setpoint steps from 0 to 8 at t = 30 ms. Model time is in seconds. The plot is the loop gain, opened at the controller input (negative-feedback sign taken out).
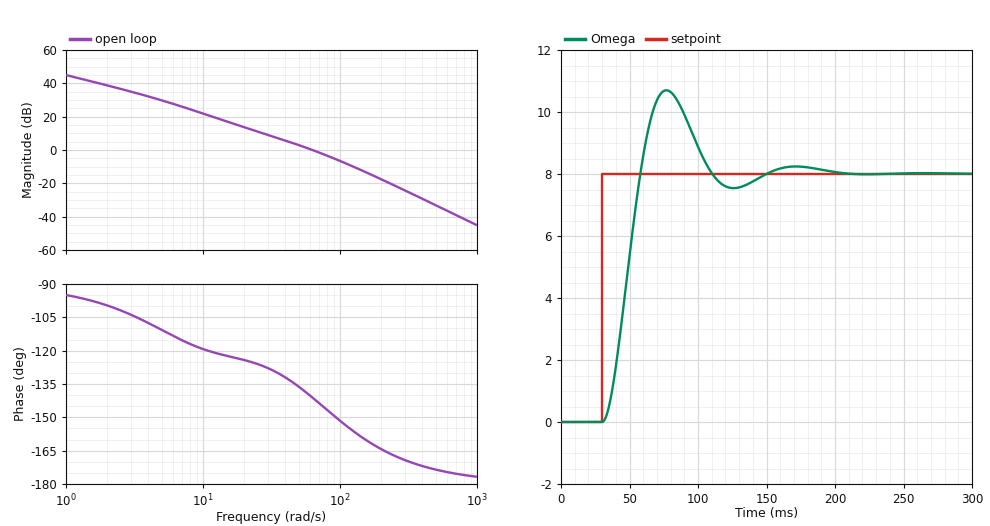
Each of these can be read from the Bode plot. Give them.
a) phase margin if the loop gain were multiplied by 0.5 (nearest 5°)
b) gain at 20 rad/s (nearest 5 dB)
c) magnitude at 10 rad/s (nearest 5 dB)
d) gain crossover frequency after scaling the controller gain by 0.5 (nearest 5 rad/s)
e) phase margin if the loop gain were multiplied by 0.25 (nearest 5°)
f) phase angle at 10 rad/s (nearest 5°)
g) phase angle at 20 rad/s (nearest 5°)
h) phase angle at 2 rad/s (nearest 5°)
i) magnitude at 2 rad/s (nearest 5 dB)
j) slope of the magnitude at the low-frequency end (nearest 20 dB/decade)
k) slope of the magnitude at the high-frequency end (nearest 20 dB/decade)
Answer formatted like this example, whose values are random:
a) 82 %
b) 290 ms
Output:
a) 50°
b) 15 dB
c) 20 dB
d) 40 rad/s
e) 55°
f) -120°
g) -125°
h) -100°
i) 40 dB
j) -20 dB/decade
k) -40 dB/decade
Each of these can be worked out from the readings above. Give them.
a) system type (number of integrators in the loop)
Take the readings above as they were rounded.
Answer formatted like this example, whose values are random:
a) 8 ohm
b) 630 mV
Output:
a) 1
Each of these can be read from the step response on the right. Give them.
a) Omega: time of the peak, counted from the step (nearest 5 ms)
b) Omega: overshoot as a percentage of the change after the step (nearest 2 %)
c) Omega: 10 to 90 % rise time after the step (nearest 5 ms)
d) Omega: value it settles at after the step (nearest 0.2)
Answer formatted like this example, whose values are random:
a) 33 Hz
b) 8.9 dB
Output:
a) 45 ms
b) 34 %
c) 20 ms
d) 8.0
